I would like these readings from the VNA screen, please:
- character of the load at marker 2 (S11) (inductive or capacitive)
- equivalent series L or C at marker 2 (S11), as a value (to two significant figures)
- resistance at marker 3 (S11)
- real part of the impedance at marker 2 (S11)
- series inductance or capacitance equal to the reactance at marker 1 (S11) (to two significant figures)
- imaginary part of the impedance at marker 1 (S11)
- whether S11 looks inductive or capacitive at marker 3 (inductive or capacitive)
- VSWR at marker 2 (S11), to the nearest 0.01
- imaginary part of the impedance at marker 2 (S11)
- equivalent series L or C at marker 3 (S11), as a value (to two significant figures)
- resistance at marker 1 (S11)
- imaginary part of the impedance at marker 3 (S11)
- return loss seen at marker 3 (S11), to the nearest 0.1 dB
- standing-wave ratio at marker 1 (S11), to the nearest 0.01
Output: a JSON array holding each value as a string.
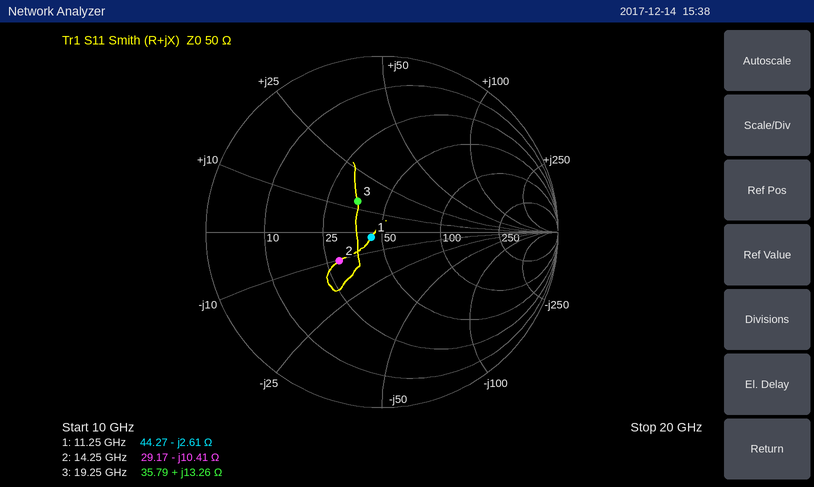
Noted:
["capacitive", "1.1 pF", "35.79 Ω", "29.17 Ω", "5.4 pF", "-2.61 Ω", "inductive", "1.82", "-10.41 Ω", "110 pH", "44.27 Ω", "+13.26 Ω", "13.0 dB", "1.14"]
